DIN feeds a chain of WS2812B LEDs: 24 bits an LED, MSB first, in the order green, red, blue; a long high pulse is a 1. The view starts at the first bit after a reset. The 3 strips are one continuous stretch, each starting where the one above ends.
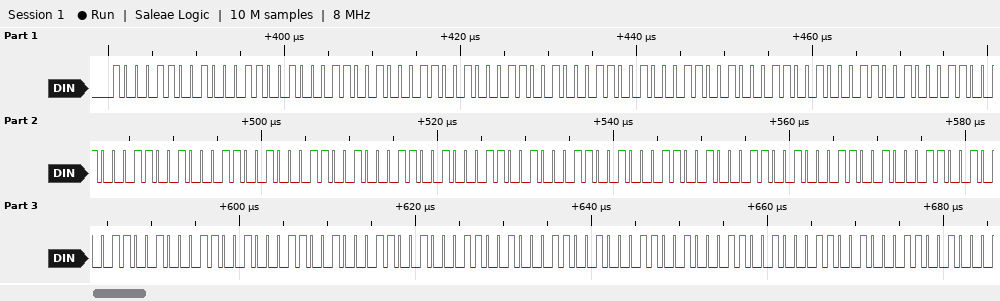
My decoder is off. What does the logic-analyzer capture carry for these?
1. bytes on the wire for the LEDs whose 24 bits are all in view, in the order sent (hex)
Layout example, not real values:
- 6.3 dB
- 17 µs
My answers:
- 8C 8C 8C 8C 8C 8C 8C 8C 8C 8C 8C 8C 8C 8C 8C 8C 8C 8C 8C 8C 8C 8C 8C 8C 8C 8C 8C 8C 8C 8C
